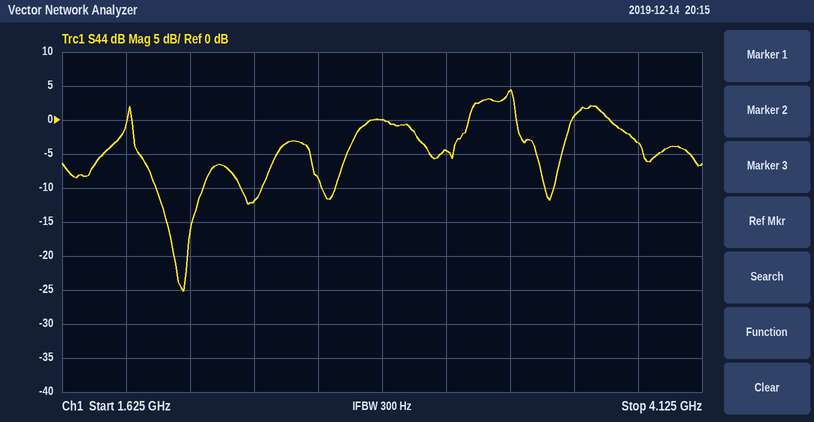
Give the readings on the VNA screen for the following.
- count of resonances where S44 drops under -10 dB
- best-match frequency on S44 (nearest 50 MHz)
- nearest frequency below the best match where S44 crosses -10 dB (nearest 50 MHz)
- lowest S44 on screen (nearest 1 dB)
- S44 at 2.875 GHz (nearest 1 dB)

4
2.10 GHz
2.00 GHz
-25 dB
0 dB
